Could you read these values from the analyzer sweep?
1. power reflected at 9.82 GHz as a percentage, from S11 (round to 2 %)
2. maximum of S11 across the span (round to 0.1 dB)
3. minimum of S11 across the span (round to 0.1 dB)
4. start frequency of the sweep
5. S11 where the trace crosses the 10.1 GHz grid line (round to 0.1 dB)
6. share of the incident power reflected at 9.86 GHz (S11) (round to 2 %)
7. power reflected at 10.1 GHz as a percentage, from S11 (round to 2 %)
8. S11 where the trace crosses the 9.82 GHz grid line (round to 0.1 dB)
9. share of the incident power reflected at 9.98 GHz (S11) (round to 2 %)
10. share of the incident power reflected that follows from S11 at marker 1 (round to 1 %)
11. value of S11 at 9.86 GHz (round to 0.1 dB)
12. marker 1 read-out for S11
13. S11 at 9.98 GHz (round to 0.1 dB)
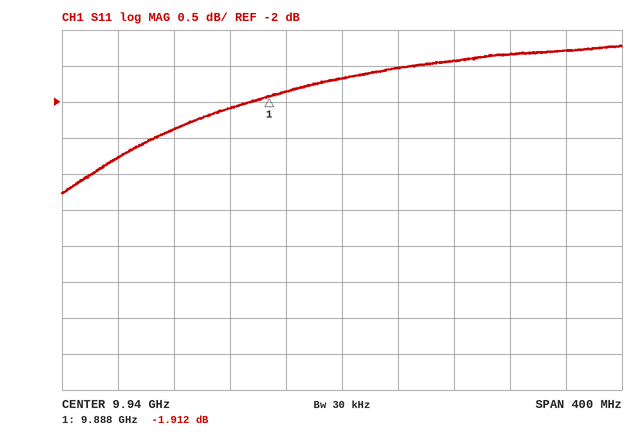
58 %
-1.2 dB
-3.3 dB
9.74 GHz
-1.3 dB
62 %
74 %
-2.4 dB
70 %
64 %
-2.1 dB
-1.912 dB
-1.5 dB
